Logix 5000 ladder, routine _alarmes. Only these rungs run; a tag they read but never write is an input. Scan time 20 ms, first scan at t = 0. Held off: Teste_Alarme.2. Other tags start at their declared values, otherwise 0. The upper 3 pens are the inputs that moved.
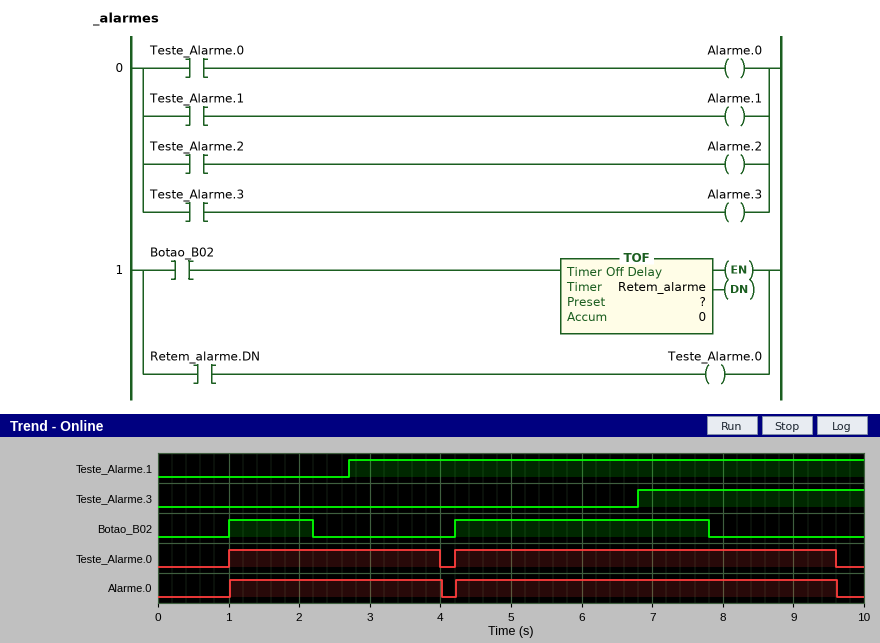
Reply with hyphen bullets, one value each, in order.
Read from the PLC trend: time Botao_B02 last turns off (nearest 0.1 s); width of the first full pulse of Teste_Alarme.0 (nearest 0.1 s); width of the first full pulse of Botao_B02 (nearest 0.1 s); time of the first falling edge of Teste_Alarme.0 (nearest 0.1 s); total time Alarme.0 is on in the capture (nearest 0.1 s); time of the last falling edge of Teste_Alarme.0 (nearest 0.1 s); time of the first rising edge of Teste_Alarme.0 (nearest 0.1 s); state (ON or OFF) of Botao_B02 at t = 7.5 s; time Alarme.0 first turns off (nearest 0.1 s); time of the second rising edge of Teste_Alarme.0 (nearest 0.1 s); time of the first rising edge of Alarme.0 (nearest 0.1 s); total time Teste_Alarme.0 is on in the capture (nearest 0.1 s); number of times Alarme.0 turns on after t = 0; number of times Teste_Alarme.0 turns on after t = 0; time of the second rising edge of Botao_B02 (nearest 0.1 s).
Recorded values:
- 7.8 s
- 3.0 s
- 1.2 s
- 4.0 s
- 8.4 s
- 9.6 s
- 1.0 s
- ON
- 4.0 s
- 4.2 s
- 1.0 s
- 8.4 s
- 2
- 2
- 4.2 s
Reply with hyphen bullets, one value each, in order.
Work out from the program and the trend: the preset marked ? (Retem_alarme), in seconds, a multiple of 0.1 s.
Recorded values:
- 1.8 s
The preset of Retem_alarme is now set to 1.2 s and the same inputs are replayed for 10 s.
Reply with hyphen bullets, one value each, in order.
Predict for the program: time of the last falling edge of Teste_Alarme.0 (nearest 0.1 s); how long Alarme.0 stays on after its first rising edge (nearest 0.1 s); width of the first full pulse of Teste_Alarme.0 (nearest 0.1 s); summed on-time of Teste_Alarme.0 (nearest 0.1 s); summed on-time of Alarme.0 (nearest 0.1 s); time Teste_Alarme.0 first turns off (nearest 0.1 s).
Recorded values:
- 9.0 s
- 2.4 s
- 2.4 s
- 7.2 s
- 7.2 s
- 3.4 s
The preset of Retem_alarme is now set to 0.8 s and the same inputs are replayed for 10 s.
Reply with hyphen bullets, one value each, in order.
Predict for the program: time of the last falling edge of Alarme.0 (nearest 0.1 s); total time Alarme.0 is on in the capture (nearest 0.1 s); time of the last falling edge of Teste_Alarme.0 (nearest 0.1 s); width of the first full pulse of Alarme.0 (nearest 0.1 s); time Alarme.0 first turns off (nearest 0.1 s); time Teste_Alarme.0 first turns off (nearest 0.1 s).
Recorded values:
- 8.6 s
- 6.4 s
- 8.6 s
- 2.0 s
- 3.0 s
- 3.0 s
